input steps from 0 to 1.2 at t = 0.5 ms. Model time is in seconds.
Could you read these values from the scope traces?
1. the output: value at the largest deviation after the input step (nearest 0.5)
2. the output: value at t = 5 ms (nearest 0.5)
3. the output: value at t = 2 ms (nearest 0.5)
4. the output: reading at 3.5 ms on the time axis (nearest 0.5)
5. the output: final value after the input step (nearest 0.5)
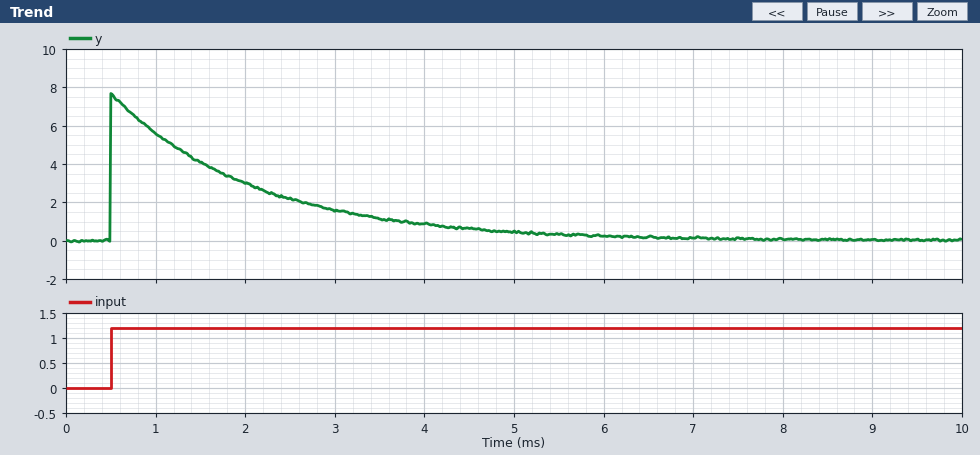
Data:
7.5
0.5
3.0
1.0
0.0
